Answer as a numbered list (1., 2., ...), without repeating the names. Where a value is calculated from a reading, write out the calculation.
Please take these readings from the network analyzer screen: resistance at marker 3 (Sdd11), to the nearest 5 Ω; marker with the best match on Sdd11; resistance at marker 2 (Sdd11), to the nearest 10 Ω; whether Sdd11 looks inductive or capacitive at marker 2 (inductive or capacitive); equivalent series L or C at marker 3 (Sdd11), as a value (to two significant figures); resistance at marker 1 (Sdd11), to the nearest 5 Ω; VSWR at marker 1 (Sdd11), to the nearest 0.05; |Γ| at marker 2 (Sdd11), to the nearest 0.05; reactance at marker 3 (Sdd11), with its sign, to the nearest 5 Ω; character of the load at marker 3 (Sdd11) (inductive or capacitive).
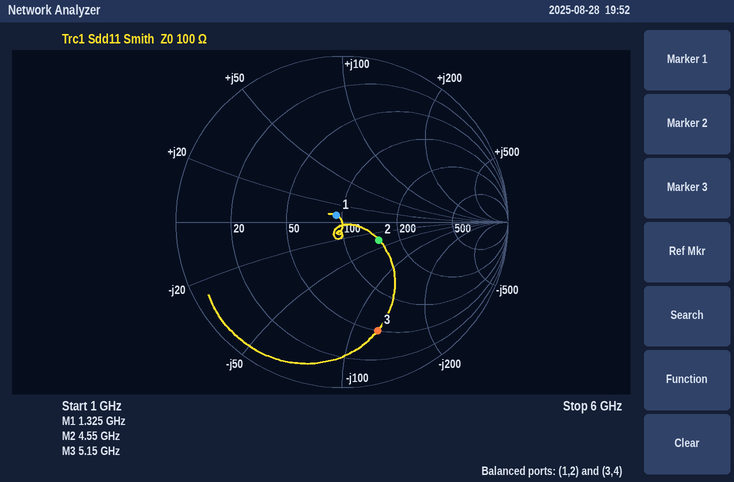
1. 50 Ω
2. marker 1
3. 150 Ω
4. capacitive
5. C = 1/(2π × 5.15 GHz × 125 Ω) ≈ 247 fF, so 250 fF to two significant figures
6. 95 Ω
7. 1.10
8. 0.25
9. -125 Ω
10. capacitive
